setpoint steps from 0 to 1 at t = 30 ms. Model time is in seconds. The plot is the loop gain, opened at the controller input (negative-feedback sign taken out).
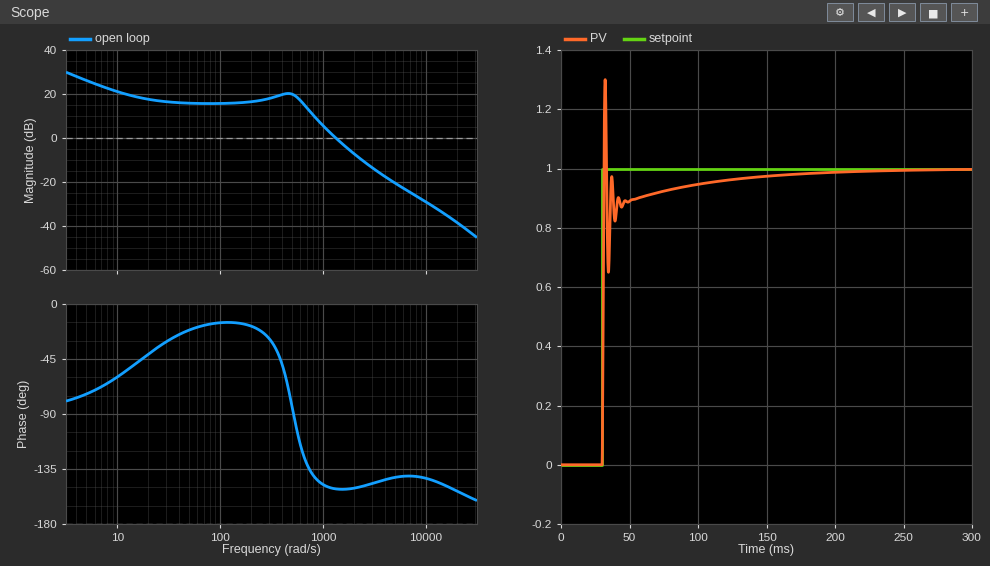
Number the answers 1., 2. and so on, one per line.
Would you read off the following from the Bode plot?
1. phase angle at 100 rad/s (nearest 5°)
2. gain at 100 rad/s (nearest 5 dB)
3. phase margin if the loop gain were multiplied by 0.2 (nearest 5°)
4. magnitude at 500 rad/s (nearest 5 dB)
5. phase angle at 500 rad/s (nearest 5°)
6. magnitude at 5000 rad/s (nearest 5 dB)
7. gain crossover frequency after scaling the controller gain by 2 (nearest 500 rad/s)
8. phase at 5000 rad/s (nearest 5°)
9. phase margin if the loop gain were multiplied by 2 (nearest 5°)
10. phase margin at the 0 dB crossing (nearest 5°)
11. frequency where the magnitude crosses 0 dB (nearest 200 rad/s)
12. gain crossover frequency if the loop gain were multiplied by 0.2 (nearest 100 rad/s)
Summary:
1. -15°
2. 15 dB
3. 50°
4. 20 dB
5. -85°
6. -20 dB
7. 2000 rad/s
8. -140°
9. 30°
10. 30°
11. 1400 rad/s
12. 700 rad/s
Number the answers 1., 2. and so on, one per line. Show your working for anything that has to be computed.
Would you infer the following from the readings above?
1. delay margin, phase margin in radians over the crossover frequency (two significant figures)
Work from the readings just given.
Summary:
1. 30 × π / 180 / 1400 = 0.00037 s
